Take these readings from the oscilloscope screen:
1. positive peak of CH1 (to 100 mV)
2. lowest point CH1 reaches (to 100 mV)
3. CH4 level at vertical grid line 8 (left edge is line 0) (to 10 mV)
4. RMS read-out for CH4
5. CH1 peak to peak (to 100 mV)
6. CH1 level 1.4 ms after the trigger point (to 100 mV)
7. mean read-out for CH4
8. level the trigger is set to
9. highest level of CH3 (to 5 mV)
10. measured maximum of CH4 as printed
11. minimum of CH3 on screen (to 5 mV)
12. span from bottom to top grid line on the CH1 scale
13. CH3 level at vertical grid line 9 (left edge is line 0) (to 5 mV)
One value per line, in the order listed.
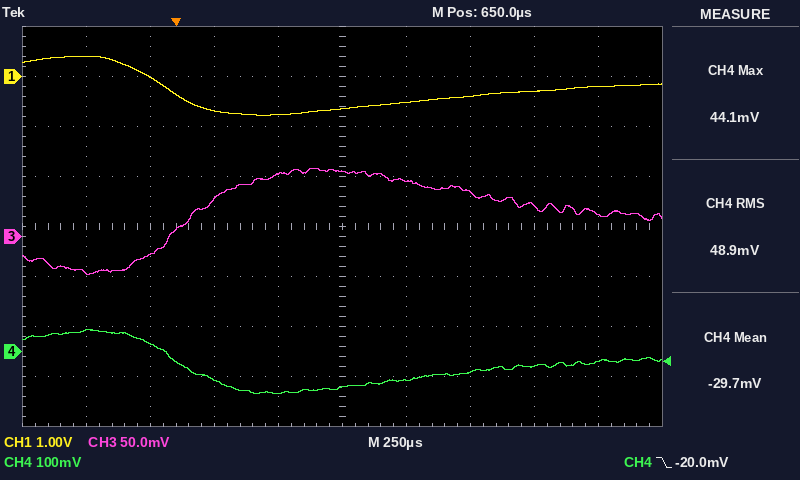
400 mV
-800 mV
-30 mV
48.9 mV
1.2 V
-300 mV
-29.7 mV
-20.0 mV
70 mV
44.1 mV
-40 mV
8 V
20 mV
